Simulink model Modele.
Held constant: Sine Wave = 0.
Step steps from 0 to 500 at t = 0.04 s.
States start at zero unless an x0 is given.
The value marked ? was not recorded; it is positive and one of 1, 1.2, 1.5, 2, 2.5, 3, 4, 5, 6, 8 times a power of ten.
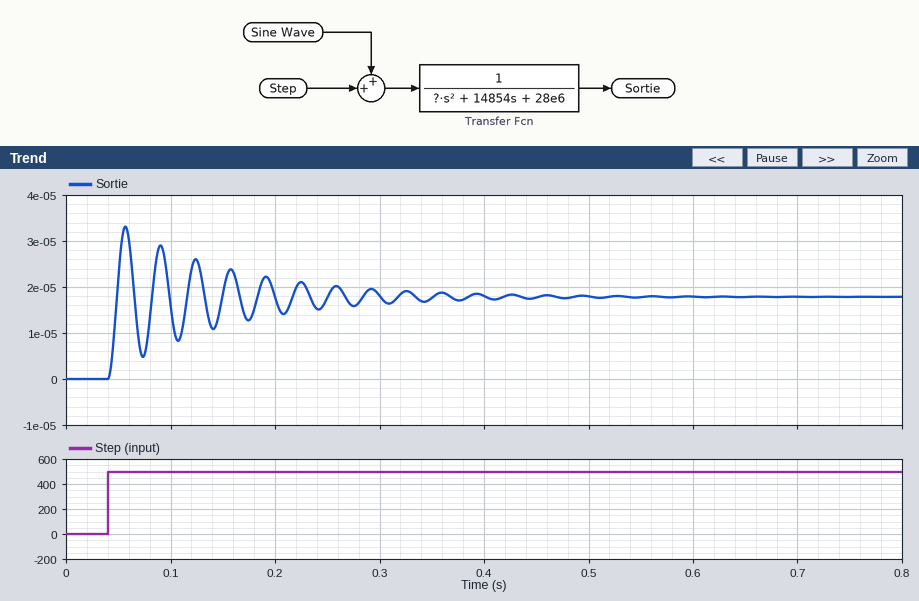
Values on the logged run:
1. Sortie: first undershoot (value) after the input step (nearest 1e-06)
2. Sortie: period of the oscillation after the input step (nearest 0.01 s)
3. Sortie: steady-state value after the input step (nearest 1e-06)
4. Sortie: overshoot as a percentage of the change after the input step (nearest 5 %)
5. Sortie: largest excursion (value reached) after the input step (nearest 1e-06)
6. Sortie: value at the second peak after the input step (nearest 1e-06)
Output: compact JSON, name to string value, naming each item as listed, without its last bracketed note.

{"Sortie: first undershoot (value) after the input step": "0.000005", "Sortie: period of the oscillation after the input step": "0.03 s", "Sortie: steady-state value after the input step": "0.000018", "Sortie: overshoot as a percentage of the change after the input step": "85 %", "Sortie: largest excursion (value reached) after the input step": "0.000033", "Sortie: value at the second peak after the input step": "0.000029"}
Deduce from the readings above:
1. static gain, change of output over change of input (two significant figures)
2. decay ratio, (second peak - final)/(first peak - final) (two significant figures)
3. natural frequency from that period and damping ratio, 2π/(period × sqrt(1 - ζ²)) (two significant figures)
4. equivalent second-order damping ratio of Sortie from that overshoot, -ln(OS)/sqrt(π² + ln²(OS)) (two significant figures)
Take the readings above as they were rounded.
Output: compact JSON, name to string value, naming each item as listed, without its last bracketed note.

{"static gain, change of output over change of input": "0.000000036", "decay ratio, (second peak - final)/(first peak - final)": "0.73", "natural frequency from that period and damping ratio, 2π/(period × sqrt(1 - ζ²))": "210 rad/s", "equivalent second-order damping ratio of Sortie from that overshoot, -ln(OS)/sqrt(π² + ln²(OS))": "0.052"}
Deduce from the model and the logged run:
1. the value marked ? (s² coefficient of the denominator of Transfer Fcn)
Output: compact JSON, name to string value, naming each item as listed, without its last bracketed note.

{"the value marked ?": "800"}
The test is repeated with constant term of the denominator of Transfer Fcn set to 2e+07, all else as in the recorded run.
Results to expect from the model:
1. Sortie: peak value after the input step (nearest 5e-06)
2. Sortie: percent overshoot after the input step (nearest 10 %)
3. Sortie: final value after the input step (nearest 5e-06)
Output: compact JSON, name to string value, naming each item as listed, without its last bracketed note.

{"Sortie: peak value after the input step": "0.000045", "Sortie: percent overshoot after the input step": "80 %", "Sortie: final value after the input step": "0.000025"}
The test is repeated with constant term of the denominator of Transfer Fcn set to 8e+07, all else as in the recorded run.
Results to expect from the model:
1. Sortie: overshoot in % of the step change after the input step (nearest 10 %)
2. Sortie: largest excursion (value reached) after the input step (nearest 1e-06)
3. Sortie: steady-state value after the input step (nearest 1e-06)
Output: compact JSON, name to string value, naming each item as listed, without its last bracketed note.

{"Sortie: overshoot in % of the step change after the input step": "90 %", "Sortie: largest excursion (value reached) after the input step": "0.000012", "Sortie: steady-state value after the input step": "0.000006"}
